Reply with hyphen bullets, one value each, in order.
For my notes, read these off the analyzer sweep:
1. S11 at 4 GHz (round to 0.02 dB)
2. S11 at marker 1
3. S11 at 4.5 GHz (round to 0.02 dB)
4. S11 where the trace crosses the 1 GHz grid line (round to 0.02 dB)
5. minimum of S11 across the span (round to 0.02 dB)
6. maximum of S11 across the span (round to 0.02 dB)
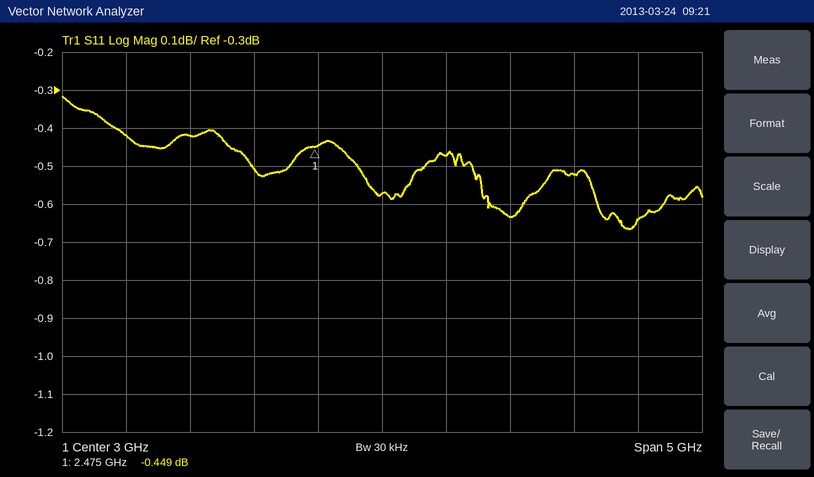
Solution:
- -0.64 dB
- -0.449 dB
- -0.52 dB
- -0.42 dB
- -0.66 dB
- -0.32 dB
